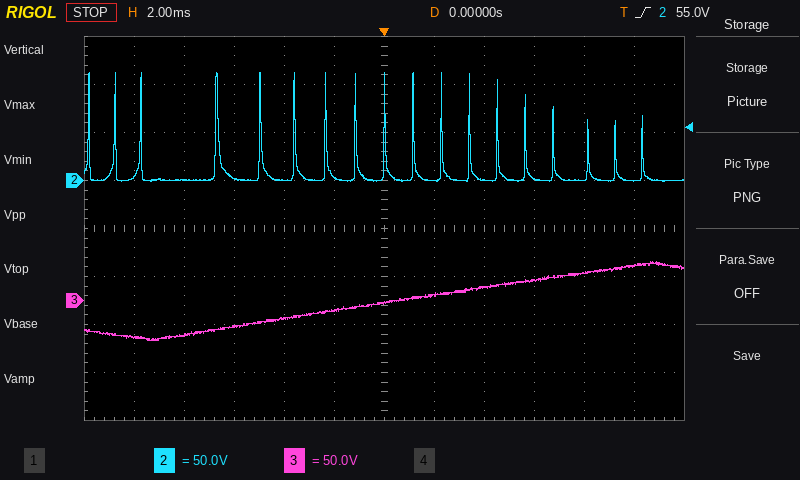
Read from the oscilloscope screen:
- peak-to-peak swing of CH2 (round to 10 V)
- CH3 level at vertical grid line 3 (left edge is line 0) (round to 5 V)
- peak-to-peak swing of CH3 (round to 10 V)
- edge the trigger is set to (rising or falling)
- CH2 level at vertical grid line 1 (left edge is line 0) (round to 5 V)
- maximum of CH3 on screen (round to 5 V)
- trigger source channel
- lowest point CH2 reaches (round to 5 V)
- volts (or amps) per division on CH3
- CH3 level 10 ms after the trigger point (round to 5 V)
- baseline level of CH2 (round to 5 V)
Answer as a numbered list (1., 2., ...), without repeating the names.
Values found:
1. 110 V
2. -25 V
3. 80 V
4. rising
5. 5 V
6. 40 V
7. CH2
8. 0 V
9. 50 V
10. 35 V
11. 0 V
